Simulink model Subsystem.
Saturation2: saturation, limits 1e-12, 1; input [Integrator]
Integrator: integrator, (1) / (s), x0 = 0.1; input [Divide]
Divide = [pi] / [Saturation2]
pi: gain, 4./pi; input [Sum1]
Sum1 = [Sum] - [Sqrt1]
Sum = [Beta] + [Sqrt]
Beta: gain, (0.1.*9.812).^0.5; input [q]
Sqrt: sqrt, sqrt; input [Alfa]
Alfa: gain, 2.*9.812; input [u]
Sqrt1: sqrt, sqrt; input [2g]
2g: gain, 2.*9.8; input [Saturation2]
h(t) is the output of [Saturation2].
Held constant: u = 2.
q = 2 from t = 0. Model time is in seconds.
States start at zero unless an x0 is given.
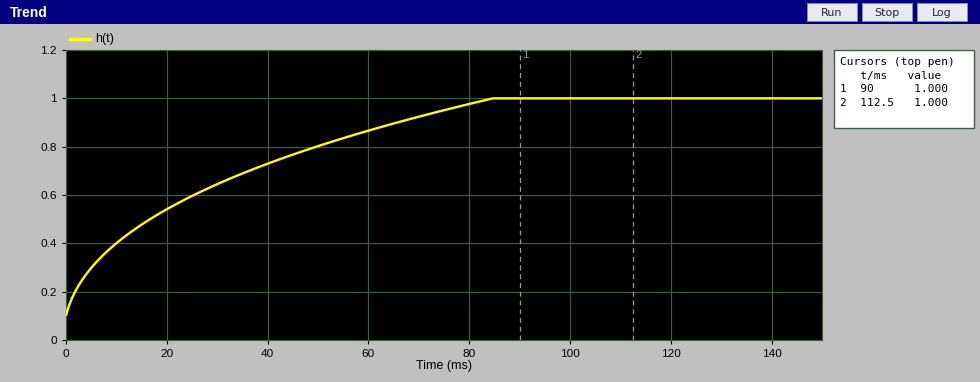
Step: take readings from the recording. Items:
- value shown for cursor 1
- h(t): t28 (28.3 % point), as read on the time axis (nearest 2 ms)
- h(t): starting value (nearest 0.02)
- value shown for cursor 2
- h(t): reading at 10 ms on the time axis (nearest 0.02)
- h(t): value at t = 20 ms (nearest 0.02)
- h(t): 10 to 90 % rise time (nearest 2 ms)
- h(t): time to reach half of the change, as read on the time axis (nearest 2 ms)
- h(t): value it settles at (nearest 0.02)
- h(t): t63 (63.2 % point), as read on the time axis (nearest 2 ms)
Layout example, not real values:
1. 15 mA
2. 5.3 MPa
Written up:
1. 1.000
2. 8 ms
3. 0.10
4. 1.000
5. 0.40
6. 0.54
7. 66 ms
8. 20 ms
9. 1.00
10. 32 ms
